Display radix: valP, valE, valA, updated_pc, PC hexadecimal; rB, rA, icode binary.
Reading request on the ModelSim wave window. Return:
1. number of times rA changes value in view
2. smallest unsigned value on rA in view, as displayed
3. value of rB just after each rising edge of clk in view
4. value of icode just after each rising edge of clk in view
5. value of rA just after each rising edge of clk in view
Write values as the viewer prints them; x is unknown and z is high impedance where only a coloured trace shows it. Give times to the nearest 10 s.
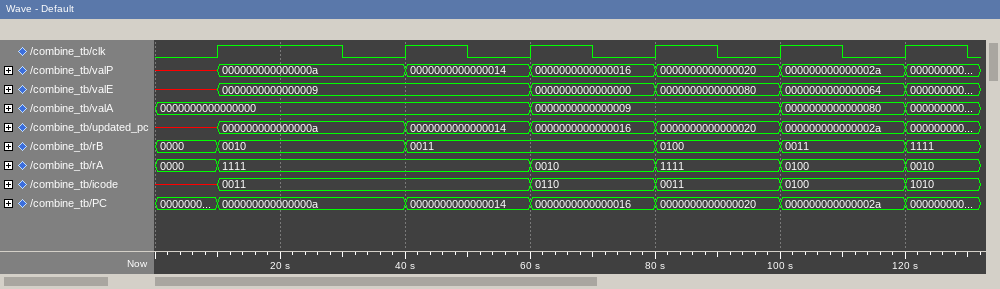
5
0000
0010, 0011, 0011, 0100, 0011, 1111
0011, 0011, 0110, 0011, 0100, 1010
1111, 1111, 0010, 1111, 0100, 0010
